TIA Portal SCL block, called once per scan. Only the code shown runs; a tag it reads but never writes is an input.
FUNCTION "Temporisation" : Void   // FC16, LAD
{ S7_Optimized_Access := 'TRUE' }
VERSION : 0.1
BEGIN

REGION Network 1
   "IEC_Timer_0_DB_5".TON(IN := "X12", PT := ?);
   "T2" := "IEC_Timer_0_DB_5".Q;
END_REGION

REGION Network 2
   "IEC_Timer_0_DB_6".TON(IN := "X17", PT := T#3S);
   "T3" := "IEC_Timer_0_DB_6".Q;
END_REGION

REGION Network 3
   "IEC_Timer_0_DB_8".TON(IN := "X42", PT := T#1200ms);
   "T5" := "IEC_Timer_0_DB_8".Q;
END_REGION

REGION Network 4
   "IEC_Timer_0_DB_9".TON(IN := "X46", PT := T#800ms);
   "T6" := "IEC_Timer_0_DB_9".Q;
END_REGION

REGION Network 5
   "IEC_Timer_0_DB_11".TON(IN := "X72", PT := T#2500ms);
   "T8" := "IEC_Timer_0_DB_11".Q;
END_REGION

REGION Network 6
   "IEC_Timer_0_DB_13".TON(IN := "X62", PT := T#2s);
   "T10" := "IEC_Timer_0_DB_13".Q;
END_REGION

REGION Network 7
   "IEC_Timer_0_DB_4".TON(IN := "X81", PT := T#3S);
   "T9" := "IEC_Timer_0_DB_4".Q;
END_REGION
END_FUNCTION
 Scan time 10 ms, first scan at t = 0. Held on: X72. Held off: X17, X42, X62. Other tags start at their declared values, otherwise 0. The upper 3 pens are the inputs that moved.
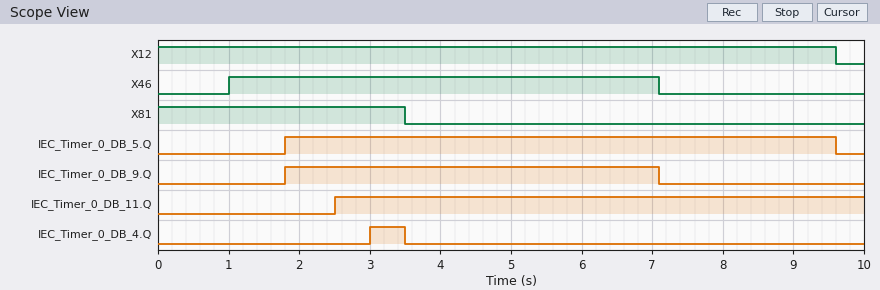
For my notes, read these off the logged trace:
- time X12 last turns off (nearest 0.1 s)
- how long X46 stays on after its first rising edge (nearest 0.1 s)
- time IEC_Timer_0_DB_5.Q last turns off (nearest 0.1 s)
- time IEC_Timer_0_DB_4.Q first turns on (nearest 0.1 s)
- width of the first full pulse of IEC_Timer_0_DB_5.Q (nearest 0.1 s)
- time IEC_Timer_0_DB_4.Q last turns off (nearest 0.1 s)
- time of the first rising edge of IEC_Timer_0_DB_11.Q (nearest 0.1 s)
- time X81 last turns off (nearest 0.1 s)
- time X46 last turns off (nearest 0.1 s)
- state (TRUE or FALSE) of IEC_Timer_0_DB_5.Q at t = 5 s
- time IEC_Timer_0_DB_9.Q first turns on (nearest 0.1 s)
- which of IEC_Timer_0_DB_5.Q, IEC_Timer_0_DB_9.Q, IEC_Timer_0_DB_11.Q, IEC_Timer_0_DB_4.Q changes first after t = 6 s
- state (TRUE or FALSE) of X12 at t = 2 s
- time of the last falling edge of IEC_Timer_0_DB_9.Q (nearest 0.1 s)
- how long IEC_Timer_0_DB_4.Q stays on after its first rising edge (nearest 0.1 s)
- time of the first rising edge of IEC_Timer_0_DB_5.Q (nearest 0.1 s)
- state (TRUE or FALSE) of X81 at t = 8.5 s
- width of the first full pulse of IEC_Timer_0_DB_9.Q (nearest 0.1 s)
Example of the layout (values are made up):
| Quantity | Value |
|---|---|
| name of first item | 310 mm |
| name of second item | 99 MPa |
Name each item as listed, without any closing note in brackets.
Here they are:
| Quantity | Value |
|---|---|
| time X12 last turns off | 9.6 s |
| how long X46 stays on after its first rising edge | 6.1 s |
| time IEC_Timer_0_DB_5.Q last turns off | 9.6 s |
| time IEC_Timer_0_DB_4.Q first turns on | 3.0 s |
| width of the first full pulse of IEC_Timer_0_DB_5.Q | 7.8 s |
| time IEC_Timer_0_DB_4.Q last turns off | 3.5 s |
| time of the first rising edge of IEC_Timer_0_DB_11.Q | 2.5 s |
| time X81 last turns off | 3.5 s |
| time X46 last turns off | 7.1 s |
| state (TRUE or FALSE) of IEC_Timer_0_DB_5.Q at t = 5 s | TRUE |
| time IEC_Timer_0_DB_9.Q first turns on | 1.8 s |
| which of IEC_Timer_0_DB_5.Q, IEC_Timer_0_DB_9.Q, IEC_Timer_0_DB_11.Q, IEC_Timer_0_DB_4.Q changes first after t = 6 s | IEC_Timer_0_DB_9.Q |
| state (TRUE or FALSE) of X12 at t = 2 s | TRUE |
| time of the last falling edge of IEC_Timer_0_DB_9.Q | 7.1 s |
| how long IEC_Timer_0_DB_4.Q stays on after its first rising edge | 0.5 s |
| time of the first rising edge of IEC_Timer_0_DB_5.Q | 1.8 s |
| state (TRUE or FALSE) of X81 at t = 8.5 s | FALSE |
| width of the first full pulse of IEC_Timer_0_DB_9.Q | 5.3 s |
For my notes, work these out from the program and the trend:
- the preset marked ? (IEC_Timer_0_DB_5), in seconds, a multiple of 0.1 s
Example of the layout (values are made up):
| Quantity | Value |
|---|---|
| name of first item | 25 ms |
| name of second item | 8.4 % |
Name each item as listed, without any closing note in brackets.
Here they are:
| Quantity | Value |
|---|---|
| the preset marked ? (IEC_Timer_0_DB_5), in seconds, a multiple of 0.1 s | 1.8 s |
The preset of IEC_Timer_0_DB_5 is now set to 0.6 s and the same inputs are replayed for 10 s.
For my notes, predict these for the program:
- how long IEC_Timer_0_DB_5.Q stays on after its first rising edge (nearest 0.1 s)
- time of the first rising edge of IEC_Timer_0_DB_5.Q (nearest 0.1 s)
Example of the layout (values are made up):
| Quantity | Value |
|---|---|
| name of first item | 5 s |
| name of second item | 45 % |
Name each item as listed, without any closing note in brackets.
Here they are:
| Quantity | Value |
|---|---|
| how long IEC_Timer_0_DB_5.Q stays on after its first rising edge | 9.0 s |
| time of the first rising edge of IEC_Timer_0_DB_5.Q | 0.6 s |
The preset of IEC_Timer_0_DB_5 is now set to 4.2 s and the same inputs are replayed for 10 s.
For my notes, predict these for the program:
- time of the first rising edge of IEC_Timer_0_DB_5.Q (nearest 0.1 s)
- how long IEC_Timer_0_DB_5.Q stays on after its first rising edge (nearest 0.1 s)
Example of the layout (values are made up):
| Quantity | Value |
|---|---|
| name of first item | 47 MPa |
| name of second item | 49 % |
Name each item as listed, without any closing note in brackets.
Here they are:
| Quantity | Value |
|---|---|
| time of the first rising edge of IEC_Timer_0_DB_5.Q | 4.2 s |
| how long IEC_Timer_0_DB_5.Q stays on after its first rising edge | 5.4 s |
